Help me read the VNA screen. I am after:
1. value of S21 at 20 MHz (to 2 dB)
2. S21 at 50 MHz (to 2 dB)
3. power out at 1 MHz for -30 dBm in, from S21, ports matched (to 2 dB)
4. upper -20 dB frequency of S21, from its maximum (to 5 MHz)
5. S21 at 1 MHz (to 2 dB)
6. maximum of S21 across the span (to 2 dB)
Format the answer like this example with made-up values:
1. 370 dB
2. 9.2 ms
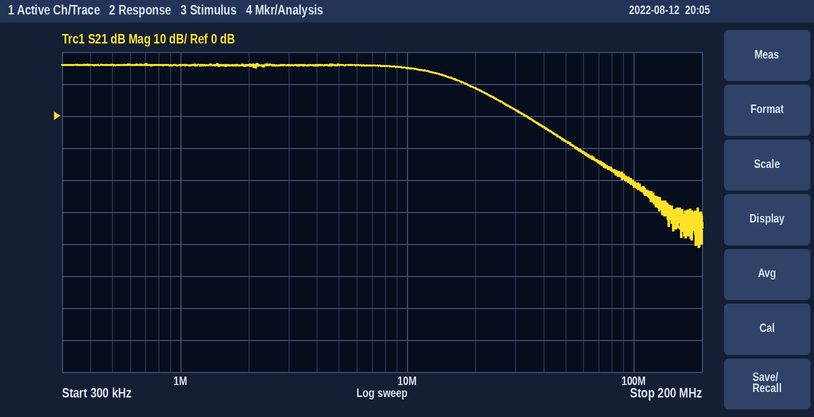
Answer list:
1. 8 dB
2. -8 dB
3. -14 dBm
4. 40 MHz
5. 16 dB
6. 16 dB
